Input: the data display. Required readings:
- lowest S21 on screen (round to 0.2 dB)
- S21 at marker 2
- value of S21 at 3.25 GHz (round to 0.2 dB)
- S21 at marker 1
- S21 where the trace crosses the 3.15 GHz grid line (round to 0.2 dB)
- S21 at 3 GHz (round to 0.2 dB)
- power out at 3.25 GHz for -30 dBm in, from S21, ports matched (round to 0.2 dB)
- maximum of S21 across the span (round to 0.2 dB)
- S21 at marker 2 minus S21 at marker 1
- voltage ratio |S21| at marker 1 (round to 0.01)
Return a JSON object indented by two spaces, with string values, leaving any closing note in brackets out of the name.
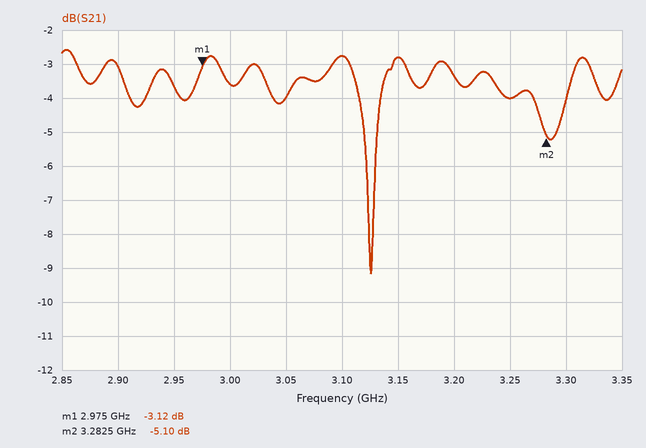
{
  "lowest S21 on screen": "-9.2 dB",
  "S21 at marker 2": "-5.10 dB",
  "value of S21 at 3.25 GHz": "-4.0 dB",
  "S21 at marker 1": "-3.12 dB",
  "S21 where the trace crosses the 3.15 GHz grid line": "-2.8 dB",
  "S21 at 3 GHz": "-3.6 dB",
  "power out at 3.25 GHz for -30 dBm in, from S21, ports matched": "-34.0 dBm",
  "maximum of S21 across the span": "-2.6 dB",
  "S21 at marker 2 minus S21 at marker 1": "-1.98 dB",
  "voltage ratio |S21| at marker 1": "0.70"
}
